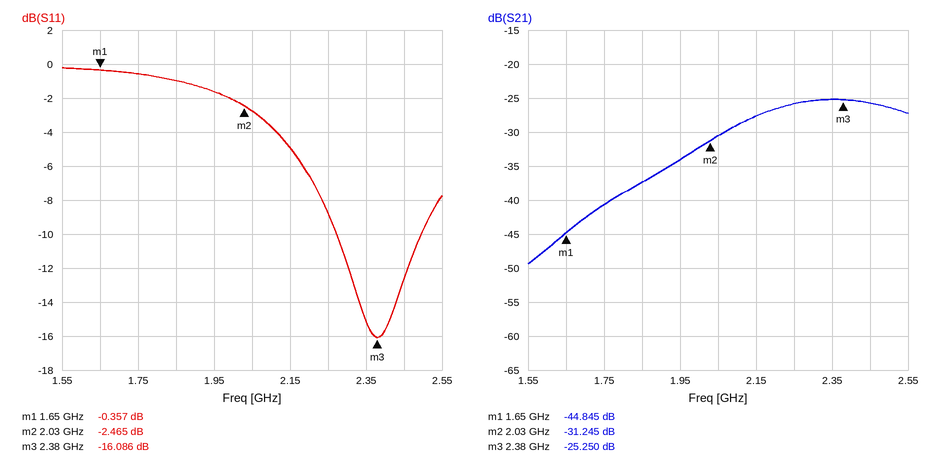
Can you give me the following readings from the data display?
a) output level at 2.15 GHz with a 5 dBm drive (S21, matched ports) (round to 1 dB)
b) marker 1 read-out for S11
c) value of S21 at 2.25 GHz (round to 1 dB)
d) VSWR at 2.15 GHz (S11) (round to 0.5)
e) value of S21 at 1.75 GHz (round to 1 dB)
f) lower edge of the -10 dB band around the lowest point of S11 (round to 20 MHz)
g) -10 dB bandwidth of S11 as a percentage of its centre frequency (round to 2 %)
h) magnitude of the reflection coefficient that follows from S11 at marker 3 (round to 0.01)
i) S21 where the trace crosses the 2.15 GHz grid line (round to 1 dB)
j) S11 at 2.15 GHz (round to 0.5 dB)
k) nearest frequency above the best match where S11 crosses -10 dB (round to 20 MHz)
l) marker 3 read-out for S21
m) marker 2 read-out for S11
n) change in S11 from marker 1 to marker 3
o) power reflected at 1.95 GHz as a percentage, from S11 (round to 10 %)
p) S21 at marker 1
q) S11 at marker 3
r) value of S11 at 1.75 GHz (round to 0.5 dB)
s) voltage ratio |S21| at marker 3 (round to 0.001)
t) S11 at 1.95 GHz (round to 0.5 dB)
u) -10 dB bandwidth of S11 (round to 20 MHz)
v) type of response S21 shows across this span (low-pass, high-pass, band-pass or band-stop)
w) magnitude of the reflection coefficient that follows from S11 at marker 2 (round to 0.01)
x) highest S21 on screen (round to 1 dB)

-23 dBm
-0.357 dB
-26 dB
3.5
-41 dB
2.28 GHz
10 %
0.16
-28 dB
-5.0 dB
2.50 GHz
-25.250 dB
-2.465 dB
-15.729 dB
70 %
-44.845 dB
-16.086 dB
-0.5 dB
0.055
-1.5 dB
220 MHz
high-pass
0.75
-25 dB
